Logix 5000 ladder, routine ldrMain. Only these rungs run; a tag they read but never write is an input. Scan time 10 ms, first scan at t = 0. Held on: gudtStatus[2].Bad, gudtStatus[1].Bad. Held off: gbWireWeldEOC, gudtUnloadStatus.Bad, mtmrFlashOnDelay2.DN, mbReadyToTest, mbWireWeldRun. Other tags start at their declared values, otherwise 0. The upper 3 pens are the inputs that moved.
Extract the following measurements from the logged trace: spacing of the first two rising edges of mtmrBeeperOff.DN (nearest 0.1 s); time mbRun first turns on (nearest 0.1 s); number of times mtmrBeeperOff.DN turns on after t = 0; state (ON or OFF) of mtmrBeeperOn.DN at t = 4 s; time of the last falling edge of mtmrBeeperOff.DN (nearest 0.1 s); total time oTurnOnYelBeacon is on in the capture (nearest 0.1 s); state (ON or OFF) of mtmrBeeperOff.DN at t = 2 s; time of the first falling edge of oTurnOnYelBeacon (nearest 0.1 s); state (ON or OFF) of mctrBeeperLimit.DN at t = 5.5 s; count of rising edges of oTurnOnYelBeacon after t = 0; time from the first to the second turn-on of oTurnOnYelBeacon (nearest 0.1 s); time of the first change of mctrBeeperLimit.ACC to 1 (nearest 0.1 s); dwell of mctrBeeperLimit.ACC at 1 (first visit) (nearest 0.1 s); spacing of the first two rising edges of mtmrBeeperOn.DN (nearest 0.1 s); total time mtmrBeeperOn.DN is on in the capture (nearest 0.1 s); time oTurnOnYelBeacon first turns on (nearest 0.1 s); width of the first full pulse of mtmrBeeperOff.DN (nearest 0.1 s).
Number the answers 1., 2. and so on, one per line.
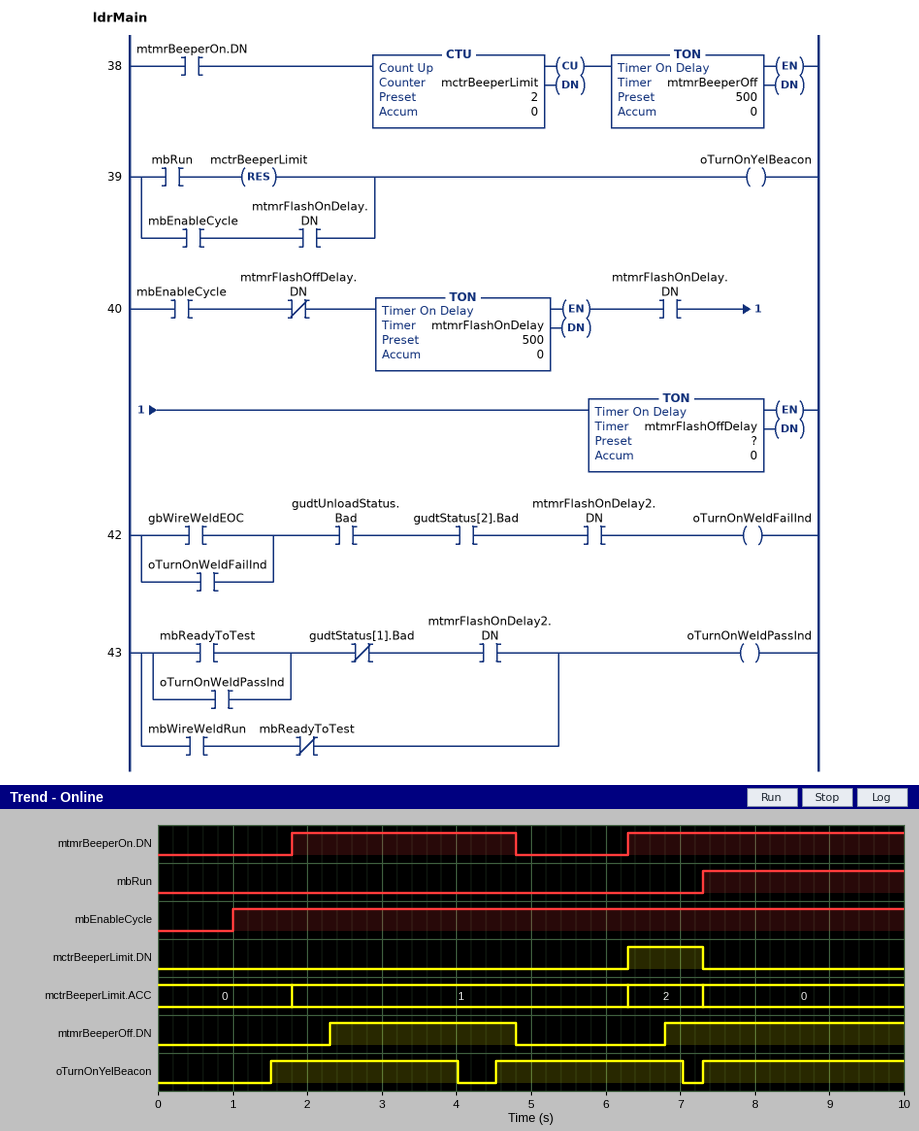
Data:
1. 4.5 s
2. 7.3 s
3. 2
4. ON
5. 4.8 s
6. 7.7 s
7. OFF
8. 4.0 s
9. OFF
10. 3
11. 3.0 s
12. 1.8 s
13. 4.5 s
14. 4.5 s
15. 6.7 s
16. 1.5 s
17. 2.5 s
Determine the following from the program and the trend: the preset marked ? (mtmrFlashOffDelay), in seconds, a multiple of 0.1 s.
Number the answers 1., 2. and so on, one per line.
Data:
1. 2.5 s
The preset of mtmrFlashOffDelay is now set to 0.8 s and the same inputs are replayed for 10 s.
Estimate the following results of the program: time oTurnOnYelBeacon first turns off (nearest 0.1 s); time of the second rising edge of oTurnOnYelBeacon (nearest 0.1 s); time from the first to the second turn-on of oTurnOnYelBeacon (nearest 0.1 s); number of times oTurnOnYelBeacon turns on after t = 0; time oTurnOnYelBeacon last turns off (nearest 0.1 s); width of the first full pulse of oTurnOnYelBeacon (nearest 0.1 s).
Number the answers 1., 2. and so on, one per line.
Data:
1. 2.3 s
2. 2.8 s
3. 1.3 s
4. 5
5. 6.3 s
6. 0.8 s
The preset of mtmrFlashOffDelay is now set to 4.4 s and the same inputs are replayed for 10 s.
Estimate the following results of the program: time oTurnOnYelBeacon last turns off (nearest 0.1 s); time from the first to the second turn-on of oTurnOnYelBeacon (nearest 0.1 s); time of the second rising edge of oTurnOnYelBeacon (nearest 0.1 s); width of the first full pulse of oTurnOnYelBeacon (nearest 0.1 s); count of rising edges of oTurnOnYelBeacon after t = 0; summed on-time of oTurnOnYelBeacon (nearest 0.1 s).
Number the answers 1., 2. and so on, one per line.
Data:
1. 5.9 s
2. 4.9 s
3. 6.4 s
4. 4.4 s
5. 2
6. 8.0 s
